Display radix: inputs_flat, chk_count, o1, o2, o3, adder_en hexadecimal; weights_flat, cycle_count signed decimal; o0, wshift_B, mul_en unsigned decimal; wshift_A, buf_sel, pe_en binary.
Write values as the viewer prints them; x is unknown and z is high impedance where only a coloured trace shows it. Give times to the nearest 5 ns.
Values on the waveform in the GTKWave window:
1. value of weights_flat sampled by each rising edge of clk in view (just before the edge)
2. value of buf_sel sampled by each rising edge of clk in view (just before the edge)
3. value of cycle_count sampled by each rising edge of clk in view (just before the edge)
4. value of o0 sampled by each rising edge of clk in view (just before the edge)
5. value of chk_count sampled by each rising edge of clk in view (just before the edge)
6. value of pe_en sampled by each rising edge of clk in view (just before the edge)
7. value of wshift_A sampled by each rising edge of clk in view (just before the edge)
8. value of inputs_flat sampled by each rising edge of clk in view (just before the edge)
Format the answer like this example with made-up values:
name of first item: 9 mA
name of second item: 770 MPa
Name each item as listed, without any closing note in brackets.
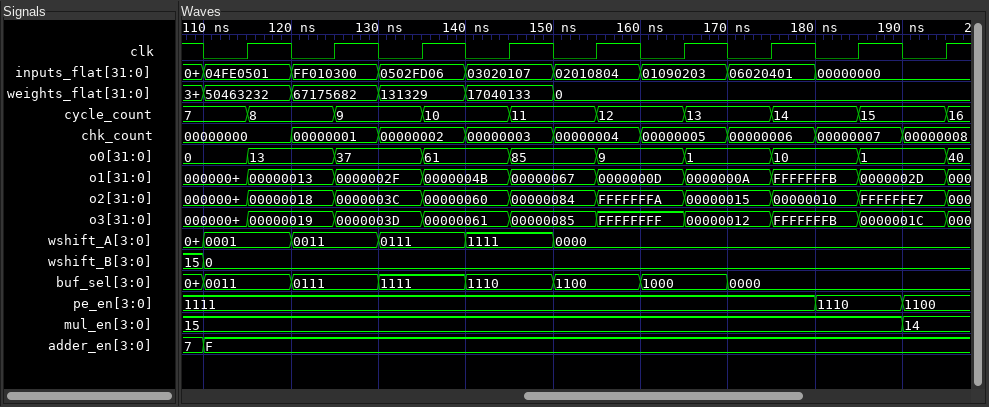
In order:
value of weights_flat sampled by each rising edge of clk in view: 50463232, 67175682, 131329, 17040133, 0, 0, 0, 0, 0
value of buf_sel sampled by each rising edge of clk in view: 0011, 0111, 1111, 1110, 1100, 1000, 0000, 0000, 0000
value of cycle_count sampled by each rising edge of clk in view: 7, 8, 9, 10, 11, 12, 13, 14, 15
value of o0 sampled by each rising edge of clk in view: 0, 13, 37, 61, 85, 9, 1, 10, 1
value of chk_count sampled by each rising edge of clk in view: 00000000, 00000001, 00000002, 00000003, 00000004, 00000005, 00000006, 00000007, 00000008
value of pe_en sampled by each rising edge of clk in view: 1111, 1111, 1111, 1111, 1111, 1111, 1111, 1110, 1100
value of wshift_A sampled by each rising edge of clk in view: 0001, 0011, 0111, 1111, 0000, 0000, 0000, 0000, 0000
value of inputs_flat sampled by each rising edge of clk in view: 04FE0501, FF010300, 0502FD06, 03020107, 02010804, 01090203, 06020401, 00000000, 00000000
